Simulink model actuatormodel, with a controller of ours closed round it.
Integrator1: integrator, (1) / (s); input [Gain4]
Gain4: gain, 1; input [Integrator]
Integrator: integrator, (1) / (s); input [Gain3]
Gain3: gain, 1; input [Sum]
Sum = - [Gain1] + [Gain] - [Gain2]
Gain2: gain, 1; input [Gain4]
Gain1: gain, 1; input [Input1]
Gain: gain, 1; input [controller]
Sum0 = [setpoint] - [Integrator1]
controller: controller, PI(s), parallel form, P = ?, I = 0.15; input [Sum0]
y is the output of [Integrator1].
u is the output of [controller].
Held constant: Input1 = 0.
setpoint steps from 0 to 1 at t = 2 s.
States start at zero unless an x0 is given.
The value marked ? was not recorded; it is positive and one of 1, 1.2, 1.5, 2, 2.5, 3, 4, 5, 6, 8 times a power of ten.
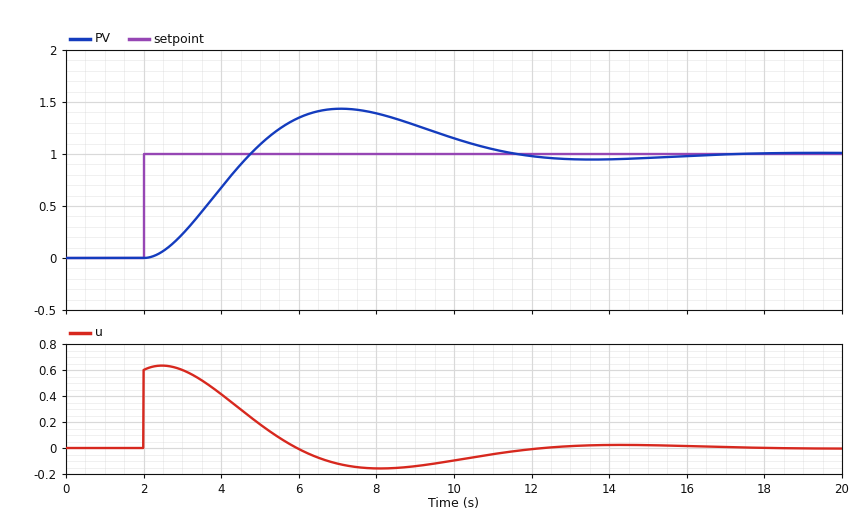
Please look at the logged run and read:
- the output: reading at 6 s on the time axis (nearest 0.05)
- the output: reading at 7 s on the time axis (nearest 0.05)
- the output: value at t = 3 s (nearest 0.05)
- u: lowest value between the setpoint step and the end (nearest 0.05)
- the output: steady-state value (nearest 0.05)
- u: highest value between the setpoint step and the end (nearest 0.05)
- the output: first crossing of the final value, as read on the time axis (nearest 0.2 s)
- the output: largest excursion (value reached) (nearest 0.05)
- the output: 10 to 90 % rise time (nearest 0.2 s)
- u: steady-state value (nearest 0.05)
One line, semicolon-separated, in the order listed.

1.35; 1.45; 0.25; -0.15; 1.00; 0.65; 4.8 s; 1.45; 1.8 s; 0.00
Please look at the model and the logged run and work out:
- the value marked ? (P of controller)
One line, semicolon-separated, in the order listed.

0.6
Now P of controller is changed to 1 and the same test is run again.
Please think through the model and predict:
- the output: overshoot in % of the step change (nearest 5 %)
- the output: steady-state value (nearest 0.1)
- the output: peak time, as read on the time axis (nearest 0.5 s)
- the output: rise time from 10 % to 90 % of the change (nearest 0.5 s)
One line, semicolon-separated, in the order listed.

35 %; 1.0; 5.5 s; 1.5 s
